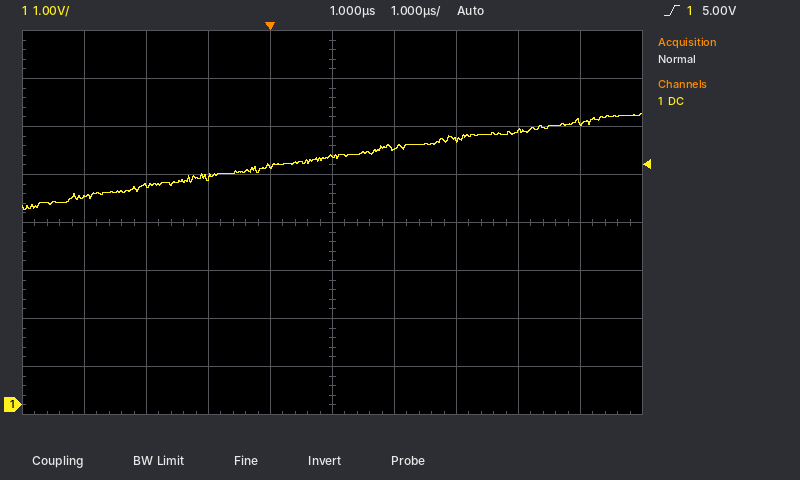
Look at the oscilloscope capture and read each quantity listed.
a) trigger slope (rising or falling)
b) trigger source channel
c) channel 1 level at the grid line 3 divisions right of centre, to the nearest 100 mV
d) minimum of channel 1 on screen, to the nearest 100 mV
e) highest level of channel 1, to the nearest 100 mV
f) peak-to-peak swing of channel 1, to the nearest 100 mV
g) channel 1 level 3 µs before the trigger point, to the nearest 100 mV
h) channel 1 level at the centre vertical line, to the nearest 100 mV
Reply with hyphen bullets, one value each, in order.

- rising
- channel 1
- 5.7 V
- 4.1 V
- 6.1 V
- 2.0 V
- 4.3 V
- 5.2 V
